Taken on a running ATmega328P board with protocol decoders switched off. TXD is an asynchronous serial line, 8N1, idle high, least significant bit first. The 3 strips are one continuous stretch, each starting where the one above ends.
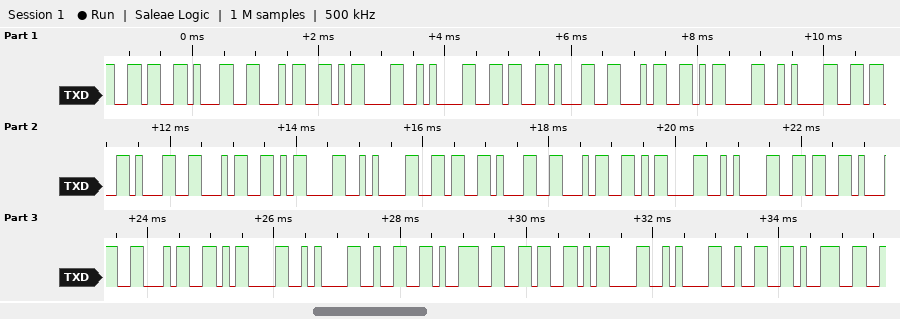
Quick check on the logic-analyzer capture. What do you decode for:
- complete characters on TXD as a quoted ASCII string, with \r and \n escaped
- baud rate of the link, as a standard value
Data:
"614\r\n614\r\n614\r\n614\r\n614\r\n296\r\n29"
9600 baud
